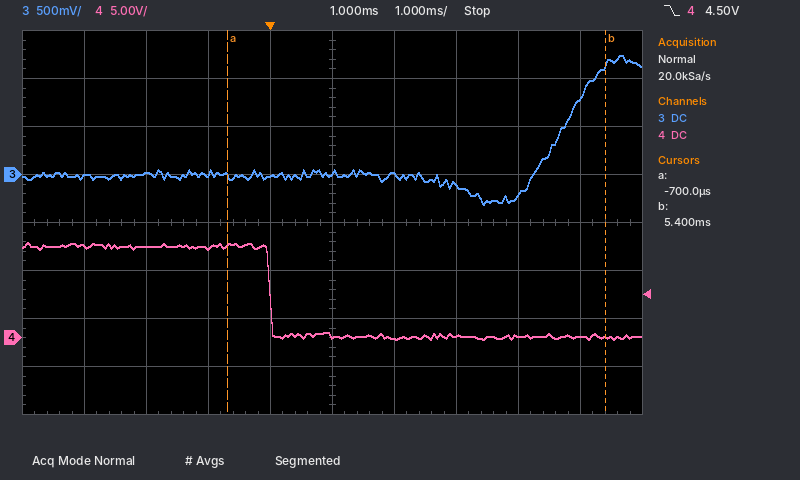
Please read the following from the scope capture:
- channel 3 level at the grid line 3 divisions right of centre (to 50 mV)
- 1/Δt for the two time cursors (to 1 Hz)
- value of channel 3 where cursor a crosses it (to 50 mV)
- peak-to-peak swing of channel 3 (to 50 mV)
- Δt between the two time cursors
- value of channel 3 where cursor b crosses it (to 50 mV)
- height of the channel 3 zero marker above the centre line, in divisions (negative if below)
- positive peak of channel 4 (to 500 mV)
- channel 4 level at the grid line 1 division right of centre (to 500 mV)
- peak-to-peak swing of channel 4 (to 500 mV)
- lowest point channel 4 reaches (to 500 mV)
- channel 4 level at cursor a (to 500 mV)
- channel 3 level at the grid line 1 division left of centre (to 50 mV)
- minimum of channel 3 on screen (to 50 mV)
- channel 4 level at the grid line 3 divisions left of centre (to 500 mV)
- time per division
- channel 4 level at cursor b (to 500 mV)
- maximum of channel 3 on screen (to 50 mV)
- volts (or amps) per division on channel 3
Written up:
-200 mV
164 Hz
0 mV
1.55 V
6.1 ms
1.15 V
+1.0 div
10.0 V
0.0 V
10.0 V
0.0 V
9.5 V
0 mV
-300 mV
9.5 V
1 ms
0.0 V
1.25 V
500 mV
